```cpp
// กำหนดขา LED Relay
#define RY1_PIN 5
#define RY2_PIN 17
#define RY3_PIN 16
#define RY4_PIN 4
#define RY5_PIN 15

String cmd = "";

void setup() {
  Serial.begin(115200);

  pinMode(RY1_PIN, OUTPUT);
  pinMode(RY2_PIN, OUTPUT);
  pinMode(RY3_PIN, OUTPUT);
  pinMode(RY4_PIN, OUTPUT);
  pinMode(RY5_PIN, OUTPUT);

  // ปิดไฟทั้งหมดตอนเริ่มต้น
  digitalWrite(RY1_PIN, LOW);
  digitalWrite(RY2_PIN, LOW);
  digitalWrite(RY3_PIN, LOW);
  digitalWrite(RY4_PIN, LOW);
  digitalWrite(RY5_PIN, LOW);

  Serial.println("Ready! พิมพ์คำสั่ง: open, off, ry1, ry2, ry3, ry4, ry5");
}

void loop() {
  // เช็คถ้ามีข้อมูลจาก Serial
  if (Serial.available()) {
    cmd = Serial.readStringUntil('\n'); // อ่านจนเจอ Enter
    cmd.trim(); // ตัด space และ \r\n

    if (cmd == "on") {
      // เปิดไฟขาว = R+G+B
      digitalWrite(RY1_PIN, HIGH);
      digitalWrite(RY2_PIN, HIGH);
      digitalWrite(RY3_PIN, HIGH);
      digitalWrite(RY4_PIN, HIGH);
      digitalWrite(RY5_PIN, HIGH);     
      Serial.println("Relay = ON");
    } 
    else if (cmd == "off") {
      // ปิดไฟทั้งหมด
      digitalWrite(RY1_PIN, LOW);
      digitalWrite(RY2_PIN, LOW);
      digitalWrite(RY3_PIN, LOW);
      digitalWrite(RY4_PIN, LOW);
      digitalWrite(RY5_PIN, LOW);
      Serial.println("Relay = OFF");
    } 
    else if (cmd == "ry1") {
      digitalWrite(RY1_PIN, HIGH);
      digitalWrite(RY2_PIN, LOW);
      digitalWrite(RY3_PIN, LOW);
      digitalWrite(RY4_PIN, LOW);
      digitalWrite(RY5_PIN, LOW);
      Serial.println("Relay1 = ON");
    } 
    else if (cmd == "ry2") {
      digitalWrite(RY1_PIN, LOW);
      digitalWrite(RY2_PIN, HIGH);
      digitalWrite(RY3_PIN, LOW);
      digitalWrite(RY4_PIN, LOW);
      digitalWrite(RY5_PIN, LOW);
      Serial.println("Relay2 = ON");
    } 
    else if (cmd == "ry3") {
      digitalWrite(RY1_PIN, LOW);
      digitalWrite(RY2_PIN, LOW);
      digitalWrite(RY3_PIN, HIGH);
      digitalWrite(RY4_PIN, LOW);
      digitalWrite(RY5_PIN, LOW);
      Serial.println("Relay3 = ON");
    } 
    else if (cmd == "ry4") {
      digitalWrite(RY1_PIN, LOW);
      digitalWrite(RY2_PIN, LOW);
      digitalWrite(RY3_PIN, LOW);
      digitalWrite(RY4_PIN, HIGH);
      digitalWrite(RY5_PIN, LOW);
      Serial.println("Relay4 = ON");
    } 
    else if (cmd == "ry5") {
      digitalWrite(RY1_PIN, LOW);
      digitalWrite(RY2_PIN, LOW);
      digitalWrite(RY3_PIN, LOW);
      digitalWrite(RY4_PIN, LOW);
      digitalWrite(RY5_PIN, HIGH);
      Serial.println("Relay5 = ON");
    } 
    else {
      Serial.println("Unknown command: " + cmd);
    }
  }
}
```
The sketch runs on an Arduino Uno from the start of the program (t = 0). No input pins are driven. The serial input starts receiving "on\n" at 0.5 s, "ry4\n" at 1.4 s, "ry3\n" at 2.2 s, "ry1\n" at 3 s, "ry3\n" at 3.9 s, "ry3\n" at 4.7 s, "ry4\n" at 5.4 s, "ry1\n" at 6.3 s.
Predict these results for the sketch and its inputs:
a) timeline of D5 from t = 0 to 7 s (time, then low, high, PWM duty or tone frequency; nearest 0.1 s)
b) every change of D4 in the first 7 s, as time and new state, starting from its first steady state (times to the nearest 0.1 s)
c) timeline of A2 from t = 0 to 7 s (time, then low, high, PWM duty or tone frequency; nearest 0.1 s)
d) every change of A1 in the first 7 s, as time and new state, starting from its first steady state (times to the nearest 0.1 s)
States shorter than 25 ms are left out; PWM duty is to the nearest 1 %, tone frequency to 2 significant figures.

0 s low; 0.5 s high; 1.4 s low; 3 s high; 3.9 s low; 6.3 s high
0 s low; 0.5 s high; 2.2 s low; 5.4 s high; 6.3 s low
0 s low; 0.5 s high; 1.4 s low; 2.2 s high; 3 s low; 3.9 s high; 5.4 s low
0 s low; 0.5 s high; 1.4 s low
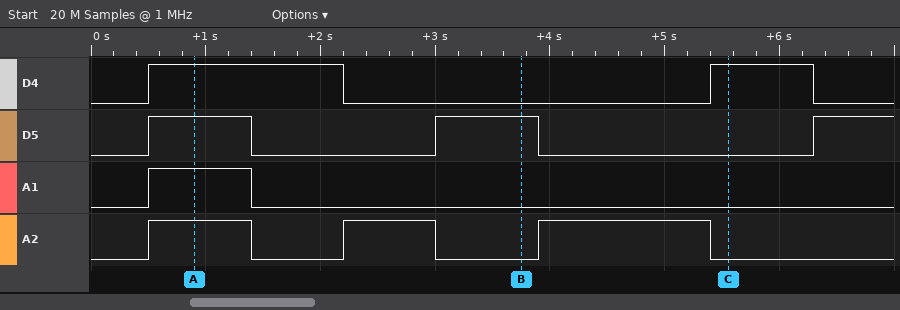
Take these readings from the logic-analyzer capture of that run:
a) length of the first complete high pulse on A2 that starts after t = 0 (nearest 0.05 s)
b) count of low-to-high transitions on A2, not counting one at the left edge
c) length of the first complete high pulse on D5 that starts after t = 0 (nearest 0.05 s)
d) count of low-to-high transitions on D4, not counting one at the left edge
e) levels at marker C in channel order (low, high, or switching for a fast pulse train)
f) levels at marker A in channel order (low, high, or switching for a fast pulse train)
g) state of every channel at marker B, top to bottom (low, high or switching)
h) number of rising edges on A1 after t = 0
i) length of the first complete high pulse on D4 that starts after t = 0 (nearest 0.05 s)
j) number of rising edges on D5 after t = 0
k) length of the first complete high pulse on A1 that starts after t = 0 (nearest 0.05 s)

0.90 s
3
0.90 s
2
D4 high, D5 low, A1 low, A2 low
D4 high, D5 high, A1 high, A2 high
D4 low, D5 high, A1 low, A2 low
1
1.70 s
3
0.90 s
